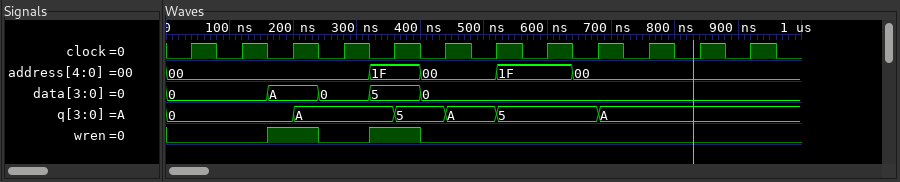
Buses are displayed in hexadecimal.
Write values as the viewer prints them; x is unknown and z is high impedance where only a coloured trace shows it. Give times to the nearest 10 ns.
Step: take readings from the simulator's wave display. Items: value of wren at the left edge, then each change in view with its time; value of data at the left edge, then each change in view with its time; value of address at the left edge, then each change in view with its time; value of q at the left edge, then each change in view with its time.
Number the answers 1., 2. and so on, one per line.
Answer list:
1. 0, 1 at 160 ns, 0 at 240 ns, 1 at 320 ns, 0 at 400 ns
2. 0, A at 160 ns, 0 at 240 ns, 5 at 320 ns, 0 at 400 ns
3. 00, 1F at 320 ns, 00 at 400 ns, 1F at 520 ns, 00 at 640 ns
4. 0, A at 200 ns, 5 at 360 ns, A at 440 ns, 5 at 520 ns, A at 680 ns
